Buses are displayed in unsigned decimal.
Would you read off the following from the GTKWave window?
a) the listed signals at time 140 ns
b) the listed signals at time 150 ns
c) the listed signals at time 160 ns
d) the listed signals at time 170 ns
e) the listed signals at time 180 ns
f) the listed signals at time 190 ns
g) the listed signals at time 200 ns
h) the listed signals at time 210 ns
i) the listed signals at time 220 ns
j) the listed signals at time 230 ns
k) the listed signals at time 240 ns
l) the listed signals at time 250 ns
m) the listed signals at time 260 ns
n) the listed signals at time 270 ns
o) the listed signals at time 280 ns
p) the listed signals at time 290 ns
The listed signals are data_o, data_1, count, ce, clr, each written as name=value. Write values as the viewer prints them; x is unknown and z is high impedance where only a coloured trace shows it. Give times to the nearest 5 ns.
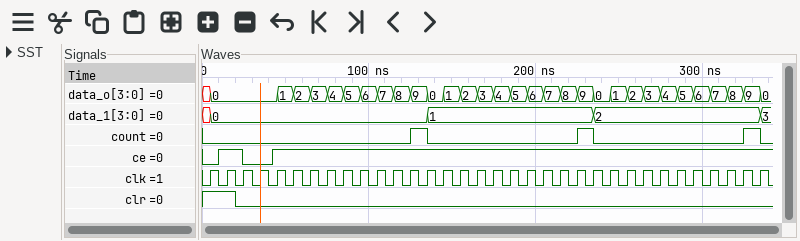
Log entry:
data_o=0, data_1=1, count=0, ce=1, clr=0
data_o=1, data_1=1, count=0, ce=1, clr=0
data_o=2, data_1=1, count=0, ce=1, clr=0
data_o=3, data_1=1, count=0, ce=1, clr=0
data_o=4, data_1=1, count=0, ce=1, clr=0
data_o=5, data_1=1, count=0, ce=1, clr=0
data_o=6, data_1=1, count=0, ce=1, clr=0
data_o=7, data_1=1, count=0, ce=1, clr=0
data_o=8, data_1=1, count=0, ce=1, clr=0
data_o=9, data_1=1, count=1, ce=1, clr=0
data_o=0, data_1=2, count=0, ce=1, clr=0
data_o=1, data_1=2, count=0, ce=1, clr=0
data_o=2, data_1=2, count=0, ce=1, clr=0
data_o=3, data_1=2, count=0, ce=1, clr=0
data_o=4, data_1=2, count=0, ce=1, clr=0
data_o=5, data_1=2, count=0, ce=1, clr=0
